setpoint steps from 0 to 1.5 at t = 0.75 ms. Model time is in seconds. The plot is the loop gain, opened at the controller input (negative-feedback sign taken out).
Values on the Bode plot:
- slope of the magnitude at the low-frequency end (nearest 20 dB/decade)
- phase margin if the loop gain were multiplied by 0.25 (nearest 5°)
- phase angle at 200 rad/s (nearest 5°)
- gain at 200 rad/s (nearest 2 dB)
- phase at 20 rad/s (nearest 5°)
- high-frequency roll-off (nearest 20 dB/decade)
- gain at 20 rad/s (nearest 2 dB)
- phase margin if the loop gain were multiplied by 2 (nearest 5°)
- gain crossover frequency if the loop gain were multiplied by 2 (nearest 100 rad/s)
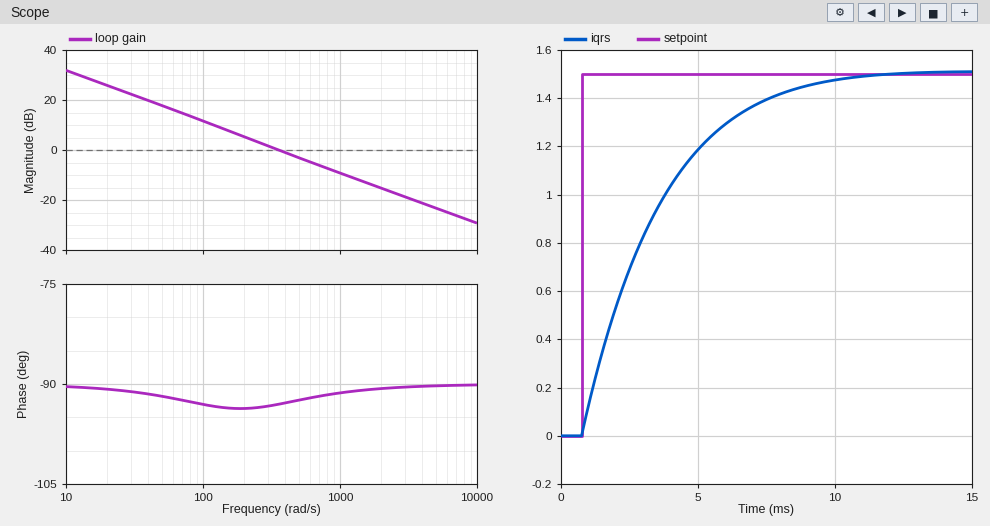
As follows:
-20 dB/decade
85°
-95°
6 dB
-90°
-20 dB/decade
26 dB
90°
700 rad/s
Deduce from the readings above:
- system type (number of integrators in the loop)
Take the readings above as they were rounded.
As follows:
1
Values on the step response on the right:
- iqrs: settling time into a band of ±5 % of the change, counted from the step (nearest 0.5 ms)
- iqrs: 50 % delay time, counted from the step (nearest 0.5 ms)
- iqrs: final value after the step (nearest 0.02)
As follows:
7.5 ms
2.0 ms
1.50
